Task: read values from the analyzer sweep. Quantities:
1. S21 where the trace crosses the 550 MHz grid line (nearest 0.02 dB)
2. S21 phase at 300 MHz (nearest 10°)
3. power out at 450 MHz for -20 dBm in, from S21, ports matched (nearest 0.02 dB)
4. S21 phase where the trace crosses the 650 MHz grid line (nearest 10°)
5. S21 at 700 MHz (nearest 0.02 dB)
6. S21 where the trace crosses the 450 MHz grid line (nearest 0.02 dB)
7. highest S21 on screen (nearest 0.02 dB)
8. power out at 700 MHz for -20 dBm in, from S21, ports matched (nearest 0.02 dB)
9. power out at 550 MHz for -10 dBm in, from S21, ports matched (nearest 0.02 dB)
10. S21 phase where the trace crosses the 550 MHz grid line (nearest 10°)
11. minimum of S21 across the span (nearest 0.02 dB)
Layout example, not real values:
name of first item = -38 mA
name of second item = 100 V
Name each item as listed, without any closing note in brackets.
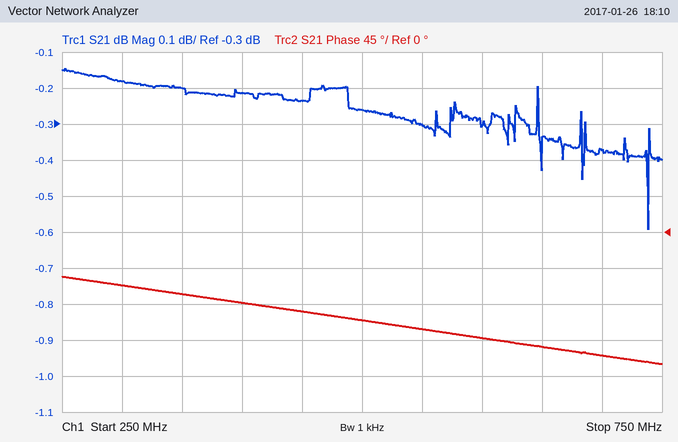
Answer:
S21 where the trace crosses the 550 MHz grid line = -0.30 dB
S21 phase at 300 MHz = -70°
power out at 450 MHz for -20 dBm in, from S21, ports matched = -20.24 dBm
S21 phase where the trace crosses the 650 MHz grid line = -140°
S21 at 700 MHz = -0.38 dB
S21 where the trace crosses the 450 MHz grid line = -0.24 dB
highest S21 on screen = -0.14 dB
power out at 700 MHz for -20 dBm in, from S21, ports matched = -20.38 dBm
power out at 550 MHz for -10 dBm in, from S21, ports matched = -10.30 dBm
S21 phase where the trace crosses the 550 MHz grid line = -120°
minimum of S21 across the span = -0.60 dB
